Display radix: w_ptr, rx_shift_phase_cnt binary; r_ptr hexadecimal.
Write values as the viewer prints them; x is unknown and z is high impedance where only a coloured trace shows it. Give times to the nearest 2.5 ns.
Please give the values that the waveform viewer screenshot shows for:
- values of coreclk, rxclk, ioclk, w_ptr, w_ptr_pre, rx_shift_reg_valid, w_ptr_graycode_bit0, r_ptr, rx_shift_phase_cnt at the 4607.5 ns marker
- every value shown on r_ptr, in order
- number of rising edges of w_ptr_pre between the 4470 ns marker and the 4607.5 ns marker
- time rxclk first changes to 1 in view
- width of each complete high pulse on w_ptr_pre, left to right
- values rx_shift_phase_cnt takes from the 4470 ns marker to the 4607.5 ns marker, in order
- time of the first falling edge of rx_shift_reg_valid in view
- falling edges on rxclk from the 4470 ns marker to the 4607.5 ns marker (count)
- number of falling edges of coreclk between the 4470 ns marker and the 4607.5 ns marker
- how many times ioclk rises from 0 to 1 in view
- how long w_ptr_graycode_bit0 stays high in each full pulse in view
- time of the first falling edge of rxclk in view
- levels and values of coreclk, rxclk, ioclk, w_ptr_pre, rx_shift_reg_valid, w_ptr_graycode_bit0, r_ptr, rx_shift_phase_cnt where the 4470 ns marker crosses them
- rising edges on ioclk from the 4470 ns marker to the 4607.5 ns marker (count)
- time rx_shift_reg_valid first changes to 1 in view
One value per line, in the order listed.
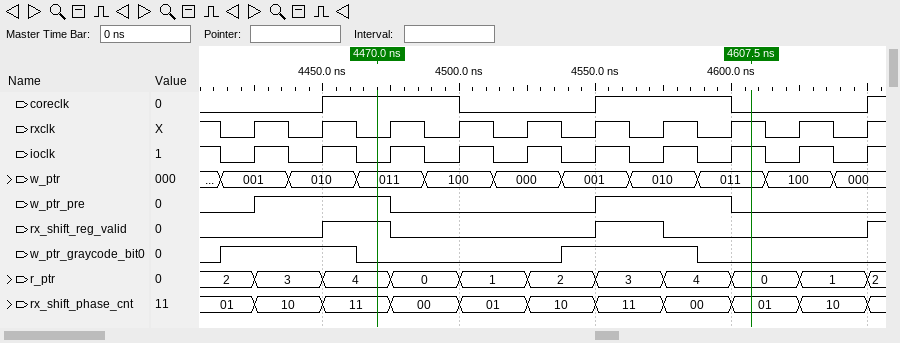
coreclk=0, rxclk=1, ioclk=1, w_ptr=011, w_ptr_pre=0, rx_shift_reg_valid=0, w_ptr_graycode_bit0=0, r_ptr=0, rx_shift_phase_cnt=01
2, 3, 4, 0, 1, 2, 3, 4, 0, 1, 2
1
4425 ns
50 ns, 50 ns
11, 00, 01, 10, 11, 00, 01
4475 ns
5
2
10
50 ns, 50 ns
4412.5 ns
coreclk=1, rxclk=0, ioclk=0, w_ptr_pre=1, rx_shift_reg_valid=1, w_ptr_graycode_bit0=0, r_ptr=4, rx_shift_phase_cnt=11
6
4450 ns
